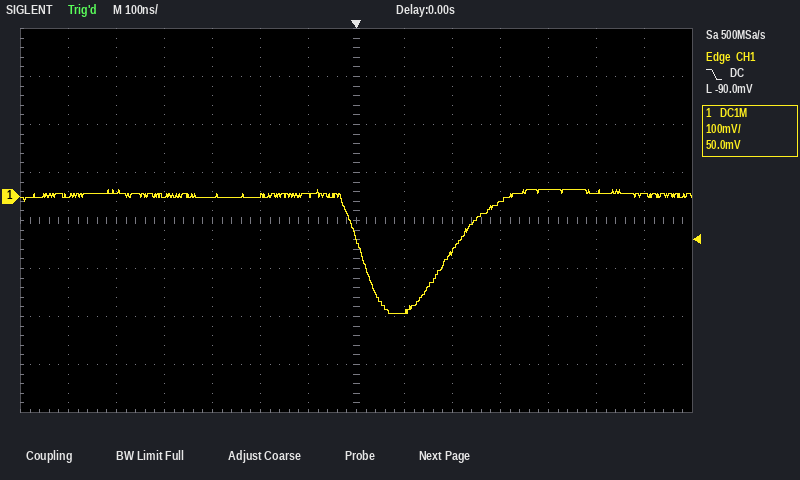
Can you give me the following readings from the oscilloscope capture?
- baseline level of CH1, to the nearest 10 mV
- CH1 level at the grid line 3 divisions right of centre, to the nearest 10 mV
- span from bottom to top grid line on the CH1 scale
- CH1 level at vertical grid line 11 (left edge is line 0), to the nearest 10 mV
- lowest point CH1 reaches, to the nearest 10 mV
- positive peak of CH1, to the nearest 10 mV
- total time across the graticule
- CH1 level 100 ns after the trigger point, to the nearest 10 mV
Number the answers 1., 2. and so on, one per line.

1. 0 mV
2. -10 mV
3. 800 mV
4. 10 mV
5. -240 mV
6. 10 mV
7. 1.4 µs
8. -240 mV
